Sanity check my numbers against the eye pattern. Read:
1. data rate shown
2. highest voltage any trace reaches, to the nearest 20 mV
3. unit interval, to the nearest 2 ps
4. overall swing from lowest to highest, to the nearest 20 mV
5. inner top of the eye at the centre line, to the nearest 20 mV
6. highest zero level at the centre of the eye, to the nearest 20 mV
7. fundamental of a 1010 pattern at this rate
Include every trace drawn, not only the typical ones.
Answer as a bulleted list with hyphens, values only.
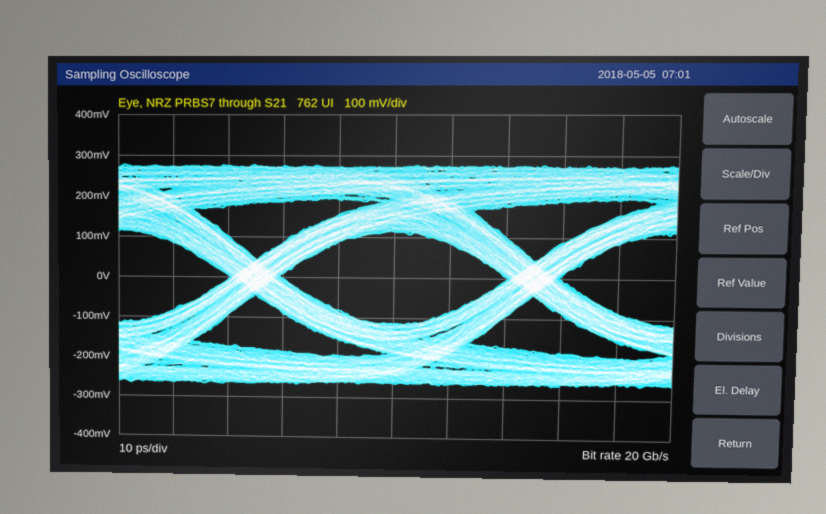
- 20 Gb/s
- 280 mV
- 50 ps
- 540 mV
- 120 mV
- -120 mV
- 10 GHz
